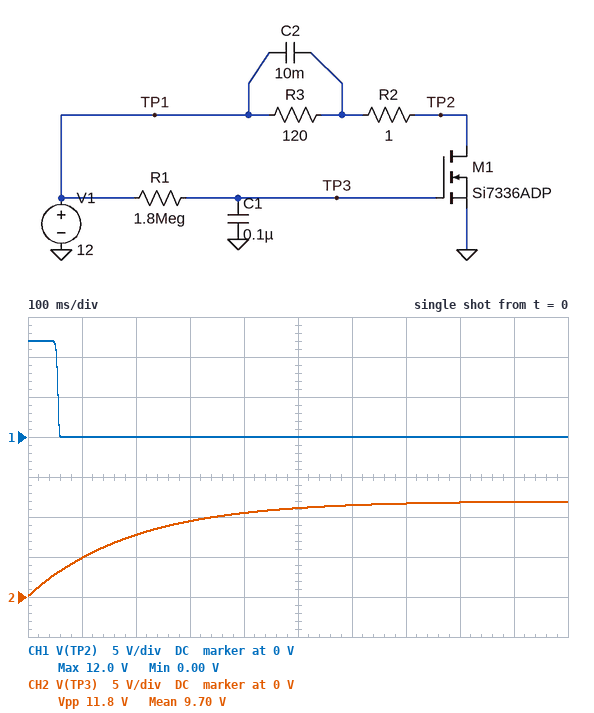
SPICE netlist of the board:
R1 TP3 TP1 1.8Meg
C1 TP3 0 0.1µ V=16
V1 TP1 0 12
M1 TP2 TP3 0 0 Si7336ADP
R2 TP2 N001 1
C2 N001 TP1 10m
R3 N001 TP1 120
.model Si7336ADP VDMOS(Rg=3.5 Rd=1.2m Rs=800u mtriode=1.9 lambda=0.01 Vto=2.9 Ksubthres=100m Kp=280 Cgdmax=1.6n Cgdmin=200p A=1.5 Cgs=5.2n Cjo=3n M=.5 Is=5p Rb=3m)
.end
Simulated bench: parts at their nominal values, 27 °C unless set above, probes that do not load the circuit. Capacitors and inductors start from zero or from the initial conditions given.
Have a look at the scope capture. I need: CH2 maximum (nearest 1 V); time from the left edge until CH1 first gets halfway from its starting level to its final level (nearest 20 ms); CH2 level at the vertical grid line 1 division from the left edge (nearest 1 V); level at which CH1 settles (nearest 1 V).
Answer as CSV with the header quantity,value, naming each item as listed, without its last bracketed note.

quantity,value
CH2 maximum,12 V
time from the left edge until CH1 first gets halfway from its starting level to its final level,60 ms
CH2 level at the vertical grid line 1 division from the left edge,5 V
level at which CH1 settles,0 V
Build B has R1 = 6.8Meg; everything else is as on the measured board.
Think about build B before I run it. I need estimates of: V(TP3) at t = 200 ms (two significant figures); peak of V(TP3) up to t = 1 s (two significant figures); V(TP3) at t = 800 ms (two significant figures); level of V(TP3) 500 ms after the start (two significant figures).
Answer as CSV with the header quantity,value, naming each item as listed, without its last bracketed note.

quantity,value
V(TP3) at t = 200 ms,3.0 V
peak of V(TP3) up to t = 1 s,9.0 V
V(TP3) at t = 800 ms,8.0 V
level of V(TP3) 500 ms after the start,6.0 V
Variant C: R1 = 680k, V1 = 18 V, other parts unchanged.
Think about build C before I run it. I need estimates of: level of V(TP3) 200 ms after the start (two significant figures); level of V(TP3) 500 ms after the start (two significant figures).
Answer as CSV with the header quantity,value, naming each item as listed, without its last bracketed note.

quantity,value
level of V(TP3) 200 ms after the start,17 V
level of V(TP3) 500 ms after the start,18 V
